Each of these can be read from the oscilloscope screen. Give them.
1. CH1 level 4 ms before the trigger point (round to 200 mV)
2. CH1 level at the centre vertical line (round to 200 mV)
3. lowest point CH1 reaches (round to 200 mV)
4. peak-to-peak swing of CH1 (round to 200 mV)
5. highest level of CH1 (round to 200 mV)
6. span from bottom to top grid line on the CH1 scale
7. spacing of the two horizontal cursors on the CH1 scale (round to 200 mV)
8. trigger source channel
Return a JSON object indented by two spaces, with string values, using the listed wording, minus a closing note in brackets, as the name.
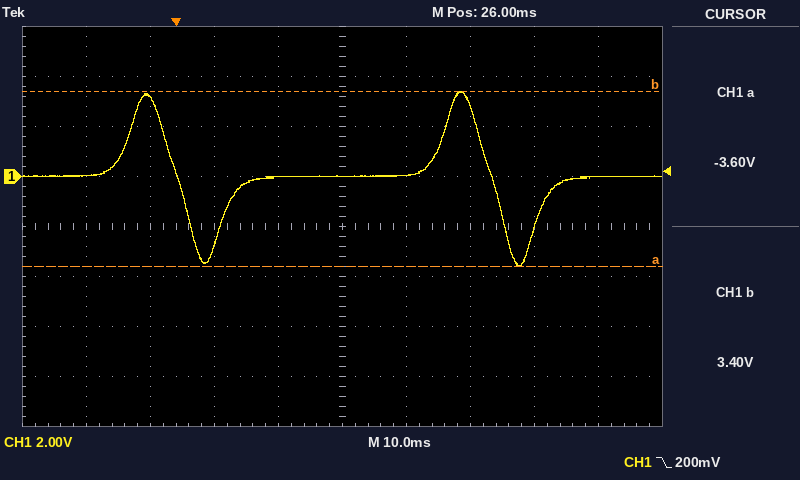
{
  "CH1 level 4 ms before the trigger point": "3.2 V",
  "CH1 level at the centre vertical line": "0.0 V",
  "lowest point CH1 reaches": "-3.6 V",
  "peak-to-peak swing of CH1": "7.0 V",
  "highest level of CH1": "3.4 V",
  "span from bottom to top grid line on the CH1 scale": "16 V",
  "spacing of the two horizontal cursors on the CH1 scale": "7.0 V",
  "trigger source channel": "CH1"
}
